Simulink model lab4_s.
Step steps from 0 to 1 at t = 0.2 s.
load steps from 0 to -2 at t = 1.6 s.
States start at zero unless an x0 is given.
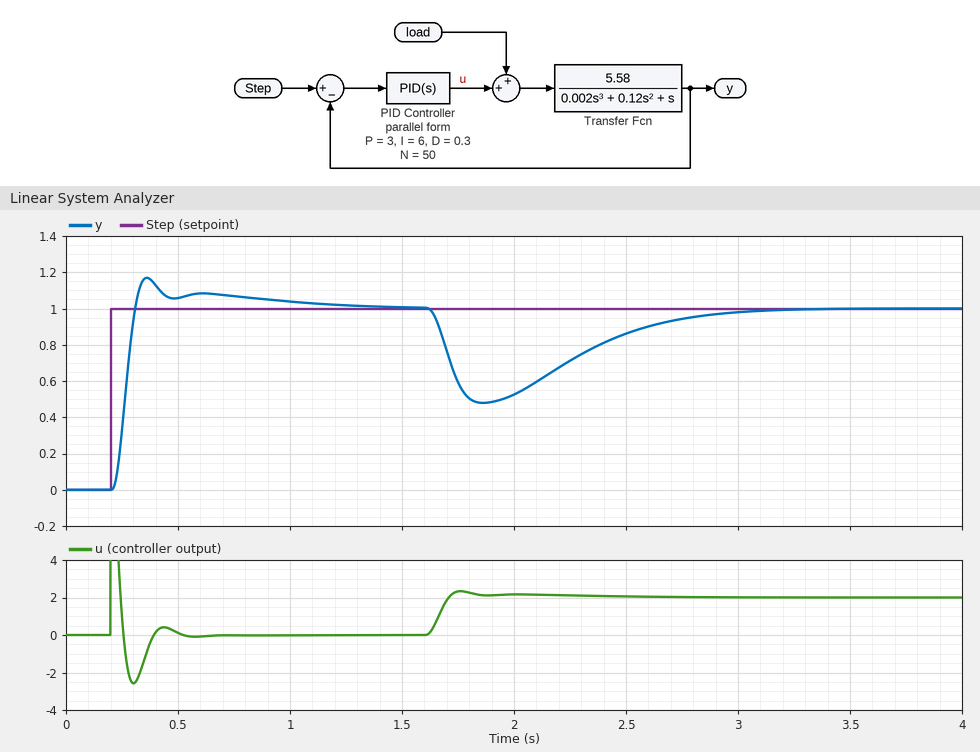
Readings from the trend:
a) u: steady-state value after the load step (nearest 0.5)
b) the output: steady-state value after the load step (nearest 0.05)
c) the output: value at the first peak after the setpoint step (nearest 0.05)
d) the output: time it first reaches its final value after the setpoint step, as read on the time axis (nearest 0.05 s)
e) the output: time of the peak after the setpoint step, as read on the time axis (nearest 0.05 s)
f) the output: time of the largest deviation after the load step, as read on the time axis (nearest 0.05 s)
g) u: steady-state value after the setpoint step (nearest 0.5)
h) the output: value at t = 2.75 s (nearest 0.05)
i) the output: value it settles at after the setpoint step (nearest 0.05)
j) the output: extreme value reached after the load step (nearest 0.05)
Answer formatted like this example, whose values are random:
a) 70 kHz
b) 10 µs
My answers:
a) 2.0
b) 1.00
c) 1.15
d) 0.30 s
e) 0.35 s
f) 1.85 s
g) 0.0
h) 0.95
i) 1.00
j) 0.50
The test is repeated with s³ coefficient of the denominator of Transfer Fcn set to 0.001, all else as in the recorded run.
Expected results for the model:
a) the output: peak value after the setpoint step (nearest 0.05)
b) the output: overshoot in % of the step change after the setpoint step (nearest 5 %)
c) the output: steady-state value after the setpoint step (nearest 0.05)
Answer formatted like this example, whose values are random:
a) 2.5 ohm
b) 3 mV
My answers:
a) 1.10
b) 10 %
c) 1.00
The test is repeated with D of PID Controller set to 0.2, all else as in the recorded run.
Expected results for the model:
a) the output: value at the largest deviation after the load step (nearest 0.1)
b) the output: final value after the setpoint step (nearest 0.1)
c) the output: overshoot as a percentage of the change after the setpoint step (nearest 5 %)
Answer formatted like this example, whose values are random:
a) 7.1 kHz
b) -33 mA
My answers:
a) 0.4
b) 1.0
c) 25 %
